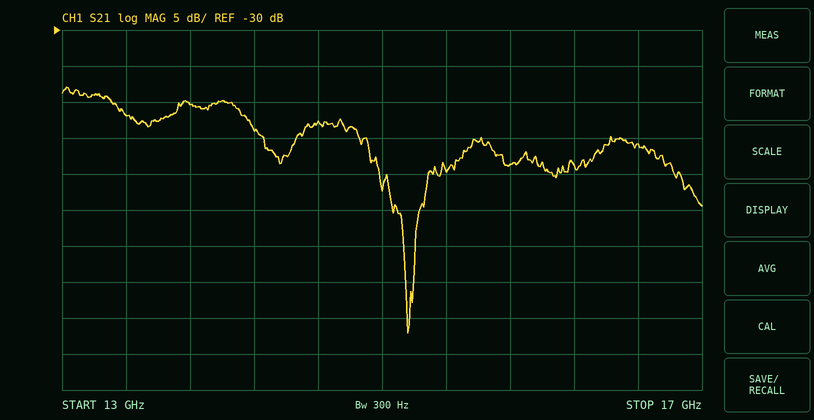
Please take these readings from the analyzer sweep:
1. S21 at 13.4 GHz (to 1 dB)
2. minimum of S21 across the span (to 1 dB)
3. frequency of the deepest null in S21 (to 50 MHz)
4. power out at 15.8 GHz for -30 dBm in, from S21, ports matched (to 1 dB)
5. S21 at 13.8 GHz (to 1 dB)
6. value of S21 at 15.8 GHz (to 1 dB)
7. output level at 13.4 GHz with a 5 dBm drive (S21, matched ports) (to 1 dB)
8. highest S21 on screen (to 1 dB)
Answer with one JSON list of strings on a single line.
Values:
["-42 dB", "-72 dB", "15.15 GHz", "-79 dBm", "-40 dB", "-49 dB", "-37 dBm", "-38 dB"]
